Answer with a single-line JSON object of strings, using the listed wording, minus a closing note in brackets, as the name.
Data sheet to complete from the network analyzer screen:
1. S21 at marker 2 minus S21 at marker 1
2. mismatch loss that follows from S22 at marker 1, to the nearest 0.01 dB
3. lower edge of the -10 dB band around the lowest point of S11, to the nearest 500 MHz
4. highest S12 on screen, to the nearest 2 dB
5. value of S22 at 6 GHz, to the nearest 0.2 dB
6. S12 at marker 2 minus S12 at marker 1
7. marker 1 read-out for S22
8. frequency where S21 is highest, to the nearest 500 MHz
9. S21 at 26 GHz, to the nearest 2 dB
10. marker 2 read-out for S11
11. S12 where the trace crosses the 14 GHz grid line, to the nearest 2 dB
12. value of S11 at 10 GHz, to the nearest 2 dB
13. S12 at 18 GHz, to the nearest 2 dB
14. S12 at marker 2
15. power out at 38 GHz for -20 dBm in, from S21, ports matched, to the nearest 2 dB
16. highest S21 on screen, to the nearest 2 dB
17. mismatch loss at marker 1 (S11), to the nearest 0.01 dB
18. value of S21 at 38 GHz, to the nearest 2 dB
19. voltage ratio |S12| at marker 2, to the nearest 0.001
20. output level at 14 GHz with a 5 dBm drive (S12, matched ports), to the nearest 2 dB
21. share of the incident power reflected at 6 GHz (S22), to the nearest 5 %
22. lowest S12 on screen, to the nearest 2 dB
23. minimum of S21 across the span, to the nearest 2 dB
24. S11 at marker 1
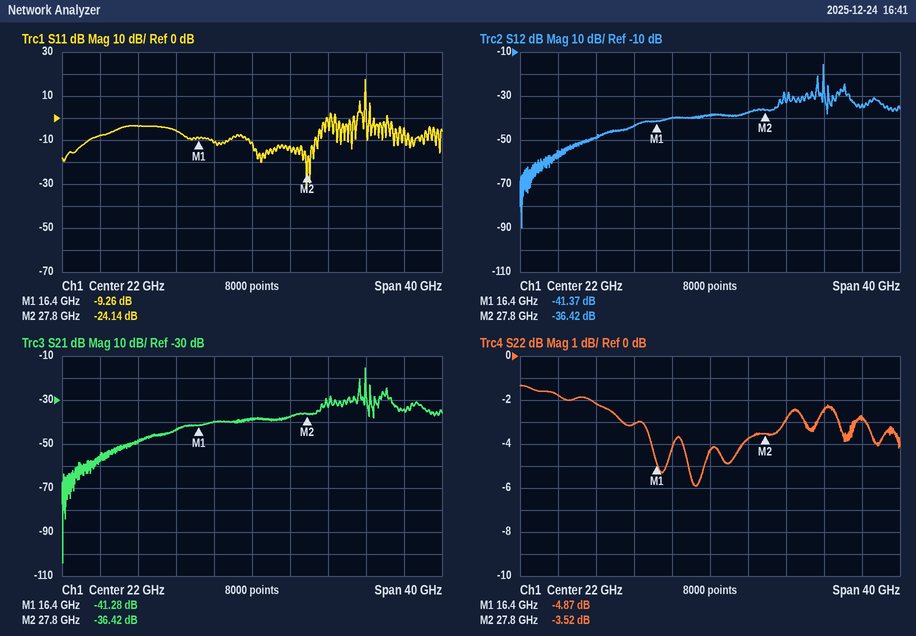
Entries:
{"S21 at marker 2 minus S21 at marker 1": "4.86 dB", "mismatch loss that follows from S22 at marker 1, to the nearest 0.01 dB": "1.71 dB", "lower edge of the -10 dB band around the lowest point of S11, to the nearest 500 MHz": "21.5 GHz", "highest S12 on screen, to the nearest 2 dB": "-16 dB", "value of S22 at 6 GHz, to the nearest 0.2 dB": "-1.8 dB", "S12 at marker 2 minus S12 at marker 1": "4.95 dB", "marker 1 read-out for S22": "-4.87 dB", "frequency where S21 is highest, to the nearest 500 MHz": "34.0 GHz", "S21 at 26 GHz, to the nearest 2 dB": "-38 dB", "marker 2 read-out for S11": "-24.14 dB", "S12 where the trace crosses the 14 GHz grid line, to the nearest 2 dB": "-44 dB", "value of S11 at 10 GHz, to the nearest 2 dB": "-4 dB", "S12 at 18 GHz, to the nearest 2 dB": "-40 dB", "S12 at marker 2": "-36.42 dB", "power out at 38 GHz for -20 dBm in, from S21, ports matched, to the nearest 2 dB": "-54 dBm", "highest S21 on screen, to the nearest 2 dB": "-16 dB", "mismatch loss at marker 1 (S11), to the nearest 0.01 dB": "0.55 dB", "value of S21 at 38 GHz, to the nearest 2 dB": "-34 dB", "voltage ratio |S12| at marker 2, to the nearest 0.001": "0.015", "output level at 14 GHz with a 5 dBm drive (S12, matched ports), to the nearest 2 dB": "-38 dBm", "share of the incident power reflected at 6 GHz (S22), to the nearest 5 %": "65 %", "lowest S12 on screen, to the nearest 2 dB": "-90 dB", "minimum of S21 across the span, to the nearest 2 dB": "-104 dB", "S11 at marker 1": "-9.26 dB"}
